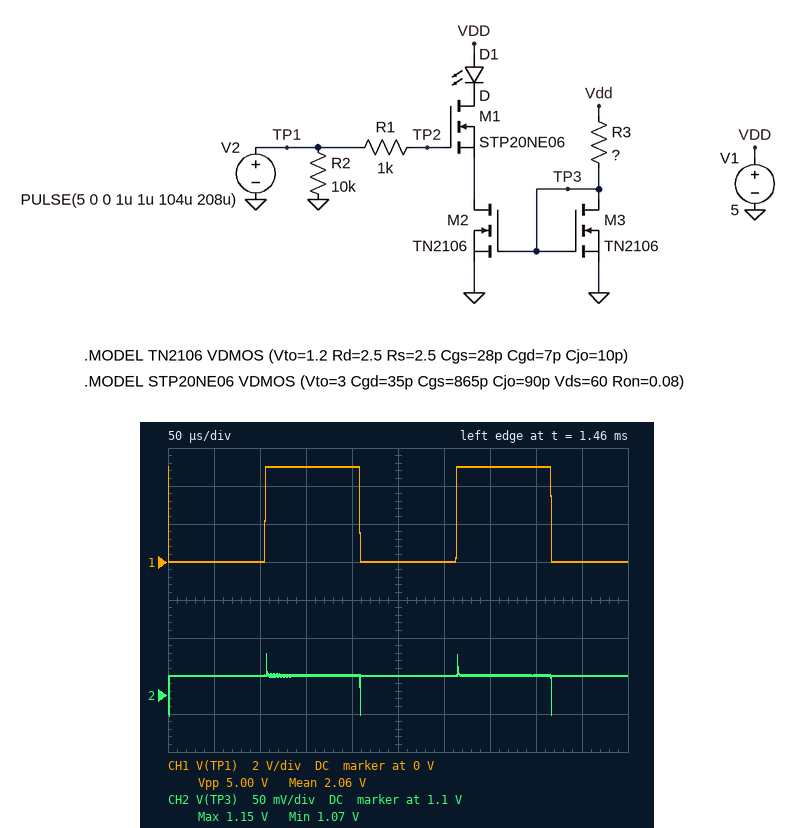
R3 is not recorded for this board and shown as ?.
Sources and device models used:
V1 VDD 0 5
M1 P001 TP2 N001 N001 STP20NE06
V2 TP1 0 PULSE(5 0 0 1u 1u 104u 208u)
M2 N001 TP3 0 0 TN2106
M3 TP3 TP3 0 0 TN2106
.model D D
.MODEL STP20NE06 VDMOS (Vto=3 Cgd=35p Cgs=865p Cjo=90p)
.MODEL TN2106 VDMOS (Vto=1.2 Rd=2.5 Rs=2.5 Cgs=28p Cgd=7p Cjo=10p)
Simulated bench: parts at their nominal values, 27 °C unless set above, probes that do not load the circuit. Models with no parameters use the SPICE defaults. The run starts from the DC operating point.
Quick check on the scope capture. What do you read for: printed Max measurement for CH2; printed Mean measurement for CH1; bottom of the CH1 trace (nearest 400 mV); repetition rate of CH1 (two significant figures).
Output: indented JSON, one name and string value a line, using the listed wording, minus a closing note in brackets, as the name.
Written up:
{
  "printed Max measurement for CH2": "1.15 V",
  "printed Mean measurement for CH1": "2.06 V",
  "bottom of the CH1 trace": "0 V",
  "repetition rate of CH1": "4.8 kHz"
}
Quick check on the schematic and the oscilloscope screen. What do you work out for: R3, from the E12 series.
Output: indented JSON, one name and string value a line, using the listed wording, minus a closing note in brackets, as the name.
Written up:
{
  "R3, from the E12 series": "270 Ω"
}
